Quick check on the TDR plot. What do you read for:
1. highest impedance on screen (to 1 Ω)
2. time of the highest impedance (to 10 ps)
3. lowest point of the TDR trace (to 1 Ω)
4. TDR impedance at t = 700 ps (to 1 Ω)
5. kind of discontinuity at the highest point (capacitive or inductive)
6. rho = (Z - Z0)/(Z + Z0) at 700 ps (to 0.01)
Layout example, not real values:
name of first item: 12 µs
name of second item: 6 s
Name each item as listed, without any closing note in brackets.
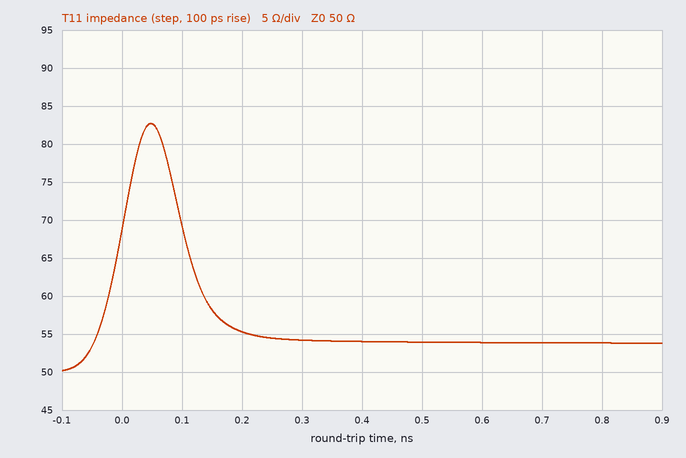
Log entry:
highest impedance on screen: 83 Ω
time of the highest impedance: 50 ps
lowest point of the TDR trace: 50 Ω
TDR impedance at t = 700 ps: 54 Ω
kind of discontinuity at the highest point: inductive
rho = (Z - Z0)/(Z + Z0) at 700 ps: +0.04
